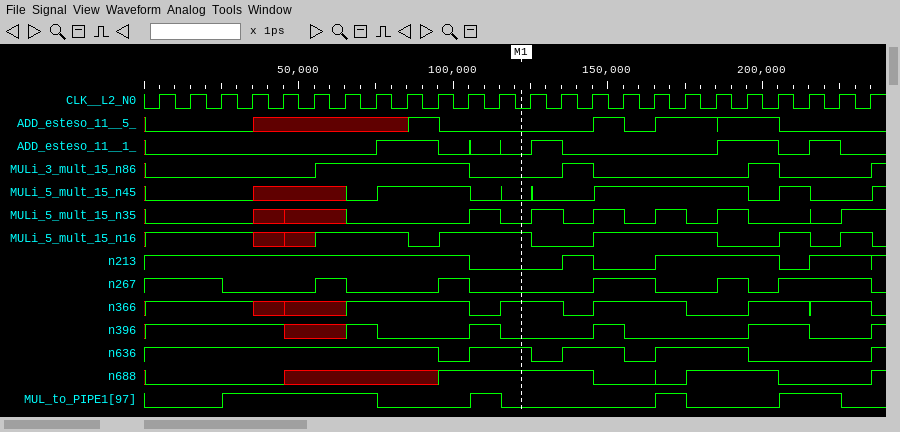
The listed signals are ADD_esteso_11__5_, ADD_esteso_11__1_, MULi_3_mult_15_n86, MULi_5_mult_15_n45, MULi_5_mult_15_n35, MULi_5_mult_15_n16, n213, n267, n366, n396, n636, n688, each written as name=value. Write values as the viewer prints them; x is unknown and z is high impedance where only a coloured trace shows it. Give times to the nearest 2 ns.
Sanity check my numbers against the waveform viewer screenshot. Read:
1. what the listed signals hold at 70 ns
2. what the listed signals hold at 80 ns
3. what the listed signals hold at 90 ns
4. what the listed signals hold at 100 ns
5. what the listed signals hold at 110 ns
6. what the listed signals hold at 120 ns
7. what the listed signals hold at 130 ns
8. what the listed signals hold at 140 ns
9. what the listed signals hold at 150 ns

ADD_esteso_11__5_=x, ADD_esteso_11__1_=0, MULi_3_mult_15_n86=1, MULi_5_mult_15_n45=0, MULi_5_mult_15_n35=0, MULi_5_mult_15_n16=1, n213=1, n267=0, n366=1, n396=1, n636=1, n688=x
ADD_esteso_11__5_=x, ADD_esteso_11__1_=1, MULi_3_mult_15_n86=1, MULi_5_mult_15_n45=1, MULi_5_mult_15_n35=0, MULi_5_mult_15_n16=1, n213=1, n267=0, n366=1, n396=0, n636=1, n688=x
ADD_esteso_11__5_=1, ADD_esteso_11__1_=1, MULi_3_mult_15_n86=1, MULi_5_mult_15_n45=1, MULi_5_mult_15_n35=0, MULi_5_mult_15_n16=0, n213=1, n267=0, n366=1, n396=0, n636=1, n688=x
ADD_esteso_11__5_=0, ADD_esteso_11__1_=0, MULi_3_mult_15_n86=1, MULi_5_mult_15_n45=1, MULi_5_mult_15_n35=0, MULi_5_mult_15_n16=1, n213=1, n267=1, n366=1, n396=0, n636=0, n688=1
ADD_esteso_11__5_=0, ADD_esteso_11__1_=0, MULi_3_mult_15_n86=0, MULi_5_mult_15_n45=0, MULi_5_mult_15_n35=1, MULi_5_mult_15_n16=1, n213=0, n267=0, n366=0, n396=1, n636=1, n688=1
ADD_esteso_11__5_=0, ADD_esteso_11__1_=0, MULi_3_mult_15_n86=0, MULi_5_mult_15_n45=0, MULi_5_mult_15_n35=0, MULi_5_mult_15_n16=1, n213=0, n267=0, n366=1, n396=0, n636=1, n688=1
ADD_esteso_11__5_=0, ADD_esteso_11__1_=1, MULi_3_mult_15_n86=0, MULi_5_mult_15_n45=0, MULi_5_mult_15_n35=1, MULi_5_mult_15_n16=0, n213=0, n267=0, n366=1, n396=0, n636=0, n688=1
ADD_esteso_11__5_=0, ADD_esteso_11__1_=0, MULi_3_mult_15_n86=1, MULi_5_mult_15_n45=0, MULi_5_mult_15_n35=0, MULi_5_mult_15_n16=0, n213=1, n267=0, n366=0, n396=0, n636=1, n688=1
ADD_esteso_11__5_=1, ADD_esteso_11__1_=0, MULi_3_mult_15_n86=0, MULi_5_mult_15_n45=1, MULi_5_mult_15_n35=1, MULi_5_mult_15_n16=1, n213=0, n267=1, n366=1, n396=1, n636=1, n688=0
